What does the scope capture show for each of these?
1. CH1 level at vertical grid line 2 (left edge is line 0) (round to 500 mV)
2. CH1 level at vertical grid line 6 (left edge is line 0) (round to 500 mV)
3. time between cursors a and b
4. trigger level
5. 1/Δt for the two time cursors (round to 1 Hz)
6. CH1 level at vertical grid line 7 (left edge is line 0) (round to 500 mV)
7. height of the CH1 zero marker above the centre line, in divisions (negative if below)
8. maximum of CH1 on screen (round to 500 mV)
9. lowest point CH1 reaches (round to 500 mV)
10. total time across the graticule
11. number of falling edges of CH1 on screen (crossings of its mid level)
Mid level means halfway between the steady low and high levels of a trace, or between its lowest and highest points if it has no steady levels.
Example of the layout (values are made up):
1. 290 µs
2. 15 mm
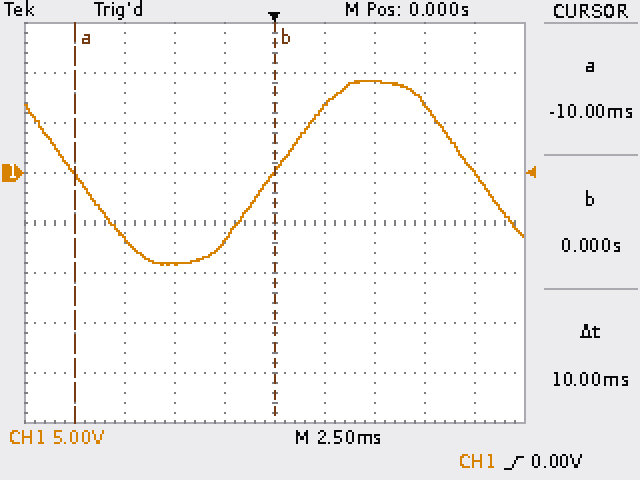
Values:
1. -6.5 V
2. 6.5 V
3. 10 ms
4. 0.00 V
5. 100 Hz
6. 9.0 V
7. +1.0 div
8. 9.0 V
9. -9.0 V
10. 25 ms
11. 2
